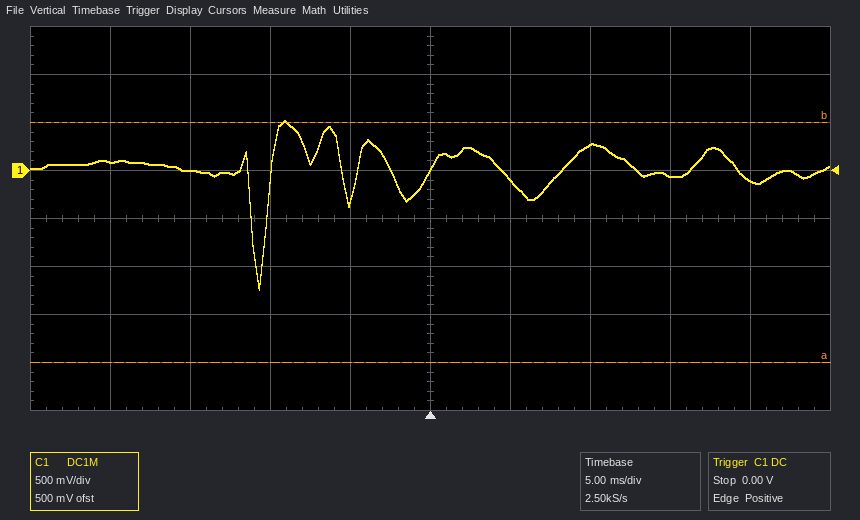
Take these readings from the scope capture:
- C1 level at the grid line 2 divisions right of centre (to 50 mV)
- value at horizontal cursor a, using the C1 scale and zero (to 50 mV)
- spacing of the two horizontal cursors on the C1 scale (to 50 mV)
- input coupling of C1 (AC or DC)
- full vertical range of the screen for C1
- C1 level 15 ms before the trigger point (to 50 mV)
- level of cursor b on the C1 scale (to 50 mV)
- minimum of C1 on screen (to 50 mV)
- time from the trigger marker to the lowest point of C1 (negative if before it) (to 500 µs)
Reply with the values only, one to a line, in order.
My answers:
250 mV
-2.00 V
2.50 V
DC
4 V
0 mV
500 mV
-1.25 V
-10.5 ms
